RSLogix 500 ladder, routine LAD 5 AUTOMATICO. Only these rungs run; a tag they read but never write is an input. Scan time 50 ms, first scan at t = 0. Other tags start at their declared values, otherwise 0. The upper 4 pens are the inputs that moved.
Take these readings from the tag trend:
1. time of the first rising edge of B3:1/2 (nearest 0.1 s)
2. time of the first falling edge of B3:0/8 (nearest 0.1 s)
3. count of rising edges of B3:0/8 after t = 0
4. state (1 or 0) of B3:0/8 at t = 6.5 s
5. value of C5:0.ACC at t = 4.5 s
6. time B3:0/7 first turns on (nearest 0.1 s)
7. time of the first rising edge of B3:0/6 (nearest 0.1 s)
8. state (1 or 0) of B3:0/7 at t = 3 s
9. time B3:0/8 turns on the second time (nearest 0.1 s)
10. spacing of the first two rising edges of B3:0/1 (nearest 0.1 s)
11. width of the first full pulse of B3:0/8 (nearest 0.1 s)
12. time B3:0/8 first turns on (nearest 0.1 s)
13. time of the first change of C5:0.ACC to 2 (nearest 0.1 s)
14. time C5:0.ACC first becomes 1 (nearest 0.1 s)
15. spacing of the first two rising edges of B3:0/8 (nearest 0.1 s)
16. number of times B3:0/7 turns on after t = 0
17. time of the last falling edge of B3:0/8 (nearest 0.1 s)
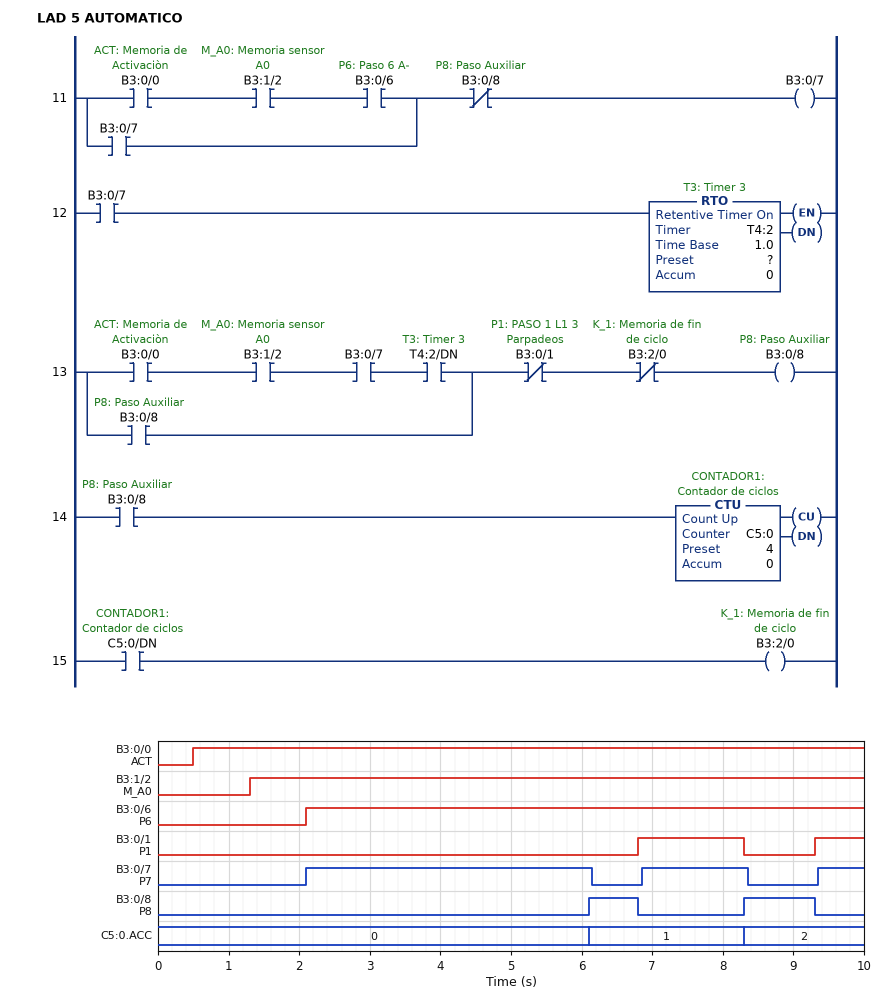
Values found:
1.3 s
6.8 s
2
1
0
2.1 s
2.1 s
1
8.3 s
2.5 s
0.7 s
6.1 s
8.3 s
6.1 s
2.2 s
3
9.3 s
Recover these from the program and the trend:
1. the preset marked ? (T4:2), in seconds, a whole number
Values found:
4 s
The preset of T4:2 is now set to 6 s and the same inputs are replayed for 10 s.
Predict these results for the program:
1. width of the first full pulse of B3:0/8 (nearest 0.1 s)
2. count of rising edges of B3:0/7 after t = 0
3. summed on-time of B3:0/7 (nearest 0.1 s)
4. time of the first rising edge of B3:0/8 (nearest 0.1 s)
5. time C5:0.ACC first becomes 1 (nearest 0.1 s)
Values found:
1.0 s
2
6.9 s
8.3 s
8.3 s
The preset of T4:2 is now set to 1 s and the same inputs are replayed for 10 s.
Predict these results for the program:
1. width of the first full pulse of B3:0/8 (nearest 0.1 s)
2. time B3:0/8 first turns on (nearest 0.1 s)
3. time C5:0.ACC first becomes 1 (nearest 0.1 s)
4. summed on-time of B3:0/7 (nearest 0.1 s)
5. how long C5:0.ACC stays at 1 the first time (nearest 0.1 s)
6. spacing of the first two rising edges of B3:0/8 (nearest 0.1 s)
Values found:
3.7 s
3.1 s
3.1 s
3.2 s
5.2 s
5.2 s
